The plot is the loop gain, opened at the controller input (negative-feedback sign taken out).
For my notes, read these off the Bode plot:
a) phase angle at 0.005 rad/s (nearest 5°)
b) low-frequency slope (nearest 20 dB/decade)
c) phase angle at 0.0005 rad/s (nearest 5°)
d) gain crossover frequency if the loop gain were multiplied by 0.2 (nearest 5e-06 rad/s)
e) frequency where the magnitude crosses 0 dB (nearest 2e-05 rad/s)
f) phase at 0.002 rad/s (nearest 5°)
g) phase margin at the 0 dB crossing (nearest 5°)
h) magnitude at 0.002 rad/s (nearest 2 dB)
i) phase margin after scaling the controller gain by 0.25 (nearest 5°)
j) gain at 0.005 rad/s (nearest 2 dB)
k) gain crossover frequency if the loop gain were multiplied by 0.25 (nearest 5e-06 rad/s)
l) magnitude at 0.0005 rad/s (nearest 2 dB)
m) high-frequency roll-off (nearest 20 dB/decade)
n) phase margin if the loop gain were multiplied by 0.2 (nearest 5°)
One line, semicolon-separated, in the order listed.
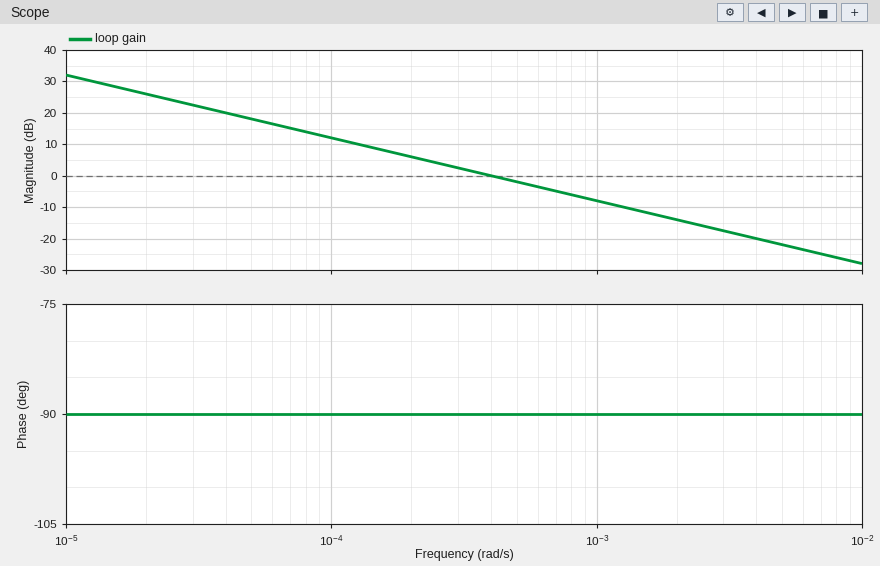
-90°; -20 dB/decade; -90°; 0.000080 rad/s; 0.00040 rad/s; -90°; 90°; -14 dB; 90°; -22 dB; 0.000100 rad/s; -2 dB; -20 dB/decade; 90°
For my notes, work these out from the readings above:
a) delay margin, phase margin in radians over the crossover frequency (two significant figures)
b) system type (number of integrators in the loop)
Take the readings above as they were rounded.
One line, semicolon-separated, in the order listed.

3900 s; 1
